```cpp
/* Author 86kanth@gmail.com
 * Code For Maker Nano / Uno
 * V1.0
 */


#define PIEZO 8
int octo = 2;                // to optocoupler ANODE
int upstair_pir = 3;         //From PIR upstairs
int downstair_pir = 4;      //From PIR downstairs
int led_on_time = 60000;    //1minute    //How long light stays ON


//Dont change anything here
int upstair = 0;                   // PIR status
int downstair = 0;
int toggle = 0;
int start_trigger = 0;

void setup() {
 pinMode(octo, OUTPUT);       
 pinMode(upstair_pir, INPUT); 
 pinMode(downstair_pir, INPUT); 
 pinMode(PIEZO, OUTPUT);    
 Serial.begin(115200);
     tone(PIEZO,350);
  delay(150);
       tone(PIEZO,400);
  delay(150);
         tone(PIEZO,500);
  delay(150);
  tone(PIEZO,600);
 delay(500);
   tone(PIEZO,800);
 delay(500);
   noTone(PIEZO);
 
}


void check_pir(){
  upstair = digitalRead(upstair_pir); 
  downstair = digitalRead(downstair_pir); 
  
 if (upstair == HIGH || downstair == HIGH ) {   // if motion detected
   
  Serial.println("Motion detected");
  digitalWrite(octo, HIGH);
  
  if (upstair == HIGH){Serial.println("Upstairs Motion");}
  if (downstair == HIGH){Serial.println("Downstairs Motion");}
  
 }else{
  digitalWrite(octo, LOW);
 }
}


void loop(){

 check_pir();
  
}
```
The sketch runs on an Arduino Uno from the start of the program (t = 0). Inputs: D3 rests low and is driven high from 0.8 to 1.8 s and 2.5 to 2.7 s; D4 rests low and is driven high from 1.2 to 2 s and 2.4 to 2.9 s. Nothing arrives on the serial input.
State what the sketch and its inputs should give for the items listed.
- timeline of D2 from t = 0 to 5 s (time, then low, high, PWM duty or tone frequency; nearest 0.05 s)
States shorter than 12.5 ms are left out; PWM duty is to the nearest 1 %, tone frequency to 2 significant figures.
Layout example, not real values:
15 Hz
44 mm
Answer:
0 s low; 1.45 s high; 2 s low; 2.4 s high; 2.9 s low
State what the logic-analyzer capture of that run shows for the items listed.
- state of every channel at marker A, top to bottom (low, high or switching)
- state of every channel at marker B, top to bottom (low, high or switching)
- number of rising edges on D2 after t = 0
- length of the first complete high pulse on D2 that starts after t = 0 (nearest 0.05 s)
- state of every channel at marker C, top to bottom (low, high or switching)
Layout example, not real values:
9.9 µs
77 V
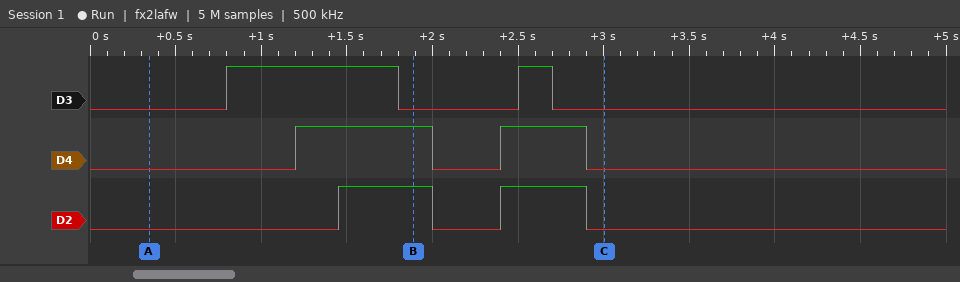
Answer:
D3 low, D4 low, D2 low
D3 low, D4 high, D2 high
2
0.55 s
D3 low, D4 low, D2 low
